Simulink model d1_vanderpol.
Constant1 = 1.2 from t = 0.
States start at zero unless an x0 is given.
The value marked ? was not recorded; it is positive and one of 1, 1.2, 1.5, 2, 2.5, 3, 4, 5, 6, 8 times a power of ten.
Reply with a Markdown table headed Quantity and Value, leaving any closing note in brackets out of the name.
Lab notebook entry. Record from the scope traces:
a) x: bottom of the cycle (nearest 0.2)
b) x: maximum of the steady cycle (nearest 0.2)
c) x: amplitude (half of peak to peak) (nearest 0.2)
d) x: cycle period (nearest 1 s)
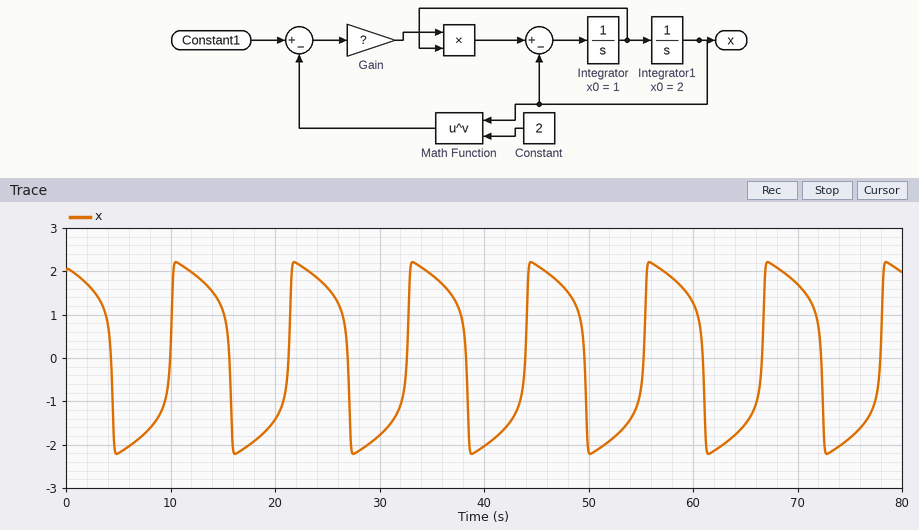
| Quantity | Value |
|---|---|
| x: bottom of the cycle | -2.2 |
| x: maximum of the steady cycle | 2.2 |
| x: amplitude (half of peak to peak) | 2.2 |
| x: cycle period | 11 s |
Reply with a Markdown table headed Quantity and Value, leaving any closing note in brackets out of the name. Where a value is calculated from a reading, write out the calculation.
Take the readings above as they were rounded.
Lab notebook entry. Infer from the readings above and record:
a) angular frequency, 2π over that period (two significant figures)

| Quantity | Value |
|---|---|
| angular frequency, 2π over that period | 2π / 11 = 0.57 rad/s |
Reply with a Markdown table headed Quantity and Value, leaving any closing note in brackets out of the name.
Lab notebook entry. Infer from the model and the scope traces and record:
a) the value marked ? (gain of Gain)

| Quantity | Value |
|---|---|
| the value marked ? | 4 |
